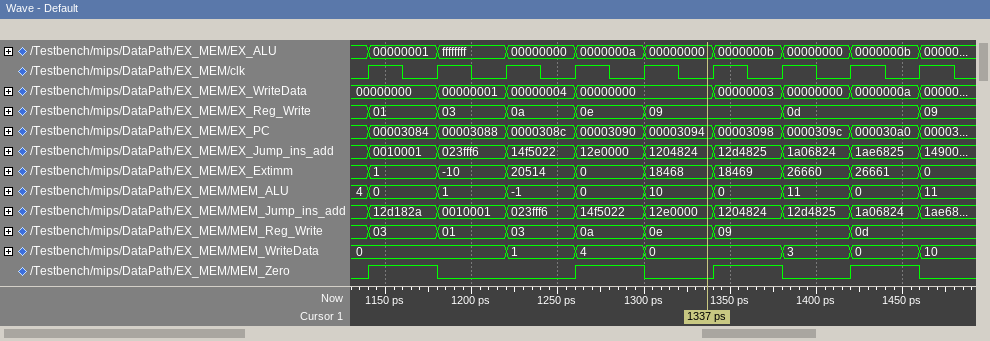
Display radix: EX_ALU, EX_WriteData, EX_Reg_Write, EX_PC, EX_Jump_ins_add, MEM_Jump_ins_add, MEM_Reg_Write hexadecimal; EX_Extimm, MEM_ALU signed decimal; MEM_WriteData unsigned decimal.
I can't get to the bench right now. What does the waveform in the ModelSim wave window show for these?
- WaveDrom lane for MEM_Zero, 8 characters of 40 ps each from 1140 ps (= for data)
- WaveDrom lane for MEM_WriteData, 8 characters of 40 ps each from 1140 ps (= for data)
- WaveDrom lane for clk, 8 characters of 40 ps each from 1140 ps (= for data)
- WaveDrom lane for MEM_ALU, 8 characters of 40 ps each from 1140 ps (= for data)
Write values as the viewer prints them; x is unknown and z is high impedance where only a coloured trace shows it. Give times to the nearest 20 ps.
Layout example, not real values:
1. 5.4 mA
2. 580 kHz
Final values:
1. {name: 'MEM_Zero', wave: '10.10101'}
2. {name: 'MEM_WriteData', wave: '=.===.==', data: '0 1 4 0 3 0'}
3. {name: 'clk', wave: 'p.......'}
4. {name: 'MEM_ALU', wave: '========', data: '0 1 -1 0 10 0 11 0'}
